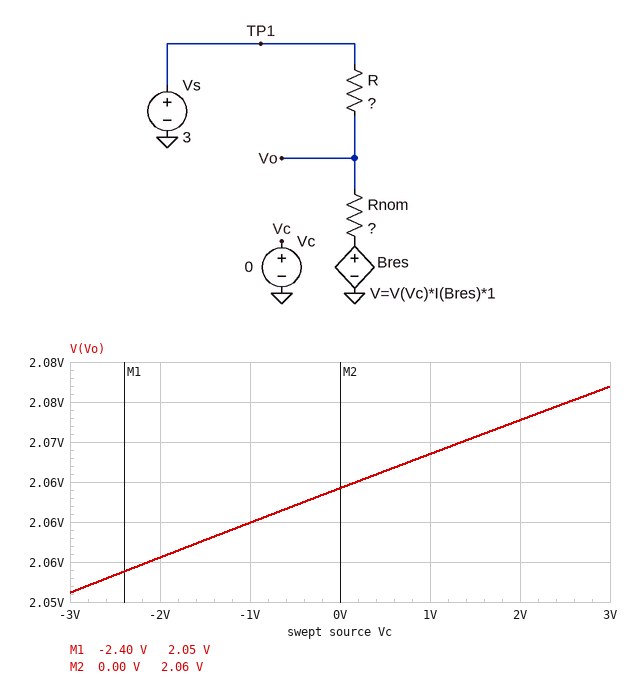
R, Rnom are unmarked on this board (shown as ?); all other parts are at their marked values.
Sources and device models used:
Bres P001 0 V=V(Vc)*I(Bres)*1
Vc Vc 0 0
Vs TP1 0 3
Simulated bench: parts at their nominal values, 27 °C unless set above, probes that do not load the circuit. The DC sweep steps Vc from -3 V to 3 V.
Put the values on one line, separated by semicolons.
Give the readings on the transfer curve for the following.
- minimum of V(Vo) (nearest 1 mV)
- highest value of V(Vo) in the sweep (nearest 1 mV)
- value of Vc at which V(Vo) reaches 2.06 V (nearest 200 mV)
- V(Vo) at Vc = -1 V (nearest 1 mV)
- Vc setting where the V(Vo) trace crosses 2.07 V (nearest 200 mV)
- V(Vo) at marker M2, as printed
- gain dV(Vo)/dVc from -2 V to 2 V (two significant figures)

2.051 V; 2.077 V; -1.0 V; 2.060 V; 1.4 V; 2.06 V; 0.0043 V/V
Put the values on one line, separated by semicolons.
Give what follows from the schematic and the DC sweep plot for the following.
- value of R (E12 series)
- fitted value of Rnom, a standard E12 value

68 Ω; 150 Ω
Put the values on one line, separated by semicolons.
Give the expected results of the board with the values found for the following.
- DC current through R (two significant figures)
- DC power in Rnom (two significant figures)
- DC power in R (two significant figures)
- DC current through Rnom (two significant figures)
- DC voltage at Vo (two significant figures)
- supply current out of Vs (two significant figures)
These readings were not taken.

14 mA; 28 mW; 13 mW; 14 mA; 2.1 V; 14 mA
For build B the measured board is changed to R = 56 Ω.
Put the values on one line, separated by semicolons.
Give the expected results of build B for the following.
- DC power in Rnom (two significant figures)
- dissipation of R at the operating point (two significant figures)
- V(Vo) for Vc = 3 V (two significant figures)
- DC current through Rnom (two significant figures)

32 mW; 12 mW; 2.2 V; 15 mA
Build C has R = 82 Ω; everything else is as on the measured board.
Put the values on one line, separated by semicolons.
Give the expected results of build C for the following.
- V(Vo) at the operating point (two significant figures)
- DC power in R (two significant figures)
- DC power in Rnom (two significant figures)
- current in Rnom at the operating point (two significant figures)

1.9 V; 14 mW; 25 mW; 13 mA
